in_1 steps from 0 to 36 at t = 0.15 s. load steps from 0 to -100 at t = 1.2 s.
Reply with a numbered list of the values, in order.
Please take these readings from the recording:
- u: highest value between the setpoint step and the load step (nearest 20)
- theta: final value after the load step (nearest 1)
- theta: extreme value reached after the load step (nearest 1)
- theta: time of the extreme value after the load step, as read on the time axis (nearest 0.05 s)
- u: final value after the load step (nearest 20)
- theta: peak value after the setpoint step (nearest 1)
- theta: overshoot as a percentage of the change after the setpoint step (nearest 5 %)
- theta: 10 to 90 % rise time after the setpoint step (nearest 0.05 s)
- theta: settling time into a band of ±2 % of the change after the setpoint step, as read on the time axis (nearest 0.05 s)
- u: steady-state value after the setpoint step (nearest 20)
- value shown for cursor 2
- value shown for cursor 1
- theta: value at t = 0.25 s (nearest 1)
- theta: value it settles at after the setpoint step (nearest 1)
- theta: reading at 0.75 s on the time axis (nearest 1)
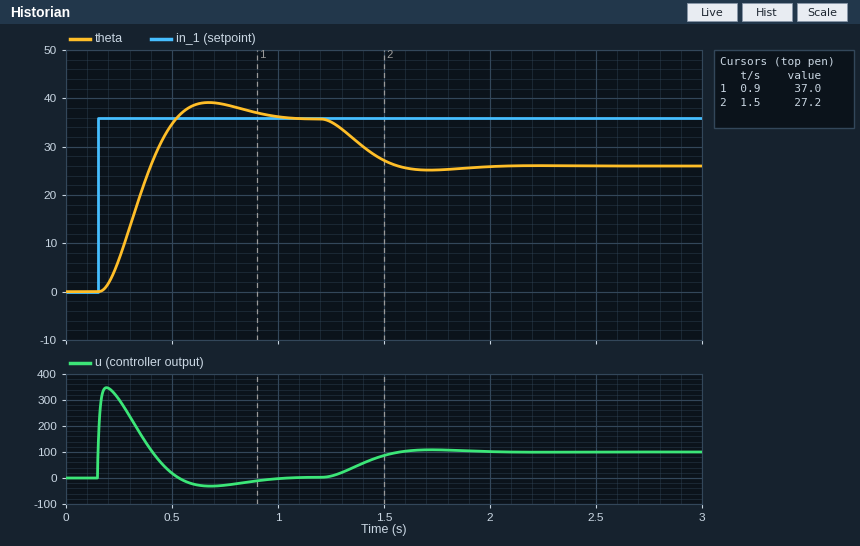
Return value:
1. 340
2. 26
3. 25
4. 1.70 s
5. 100
6. 39
7. 10 %
8. 0.25 s
9. 0.95 s
10. 0
11. 27.2
12. 37.0
13. 7
14. 36
15. 39
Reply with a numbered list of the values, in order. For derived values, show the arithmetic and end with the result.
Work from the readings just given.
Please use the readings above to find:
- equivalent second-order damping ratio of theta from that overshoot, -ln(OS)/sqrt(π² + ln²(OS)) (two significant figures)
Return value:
1. ln(0.1) = -2.303; 2.303 / sqrt(9.870 + 5.302) = 0.59
